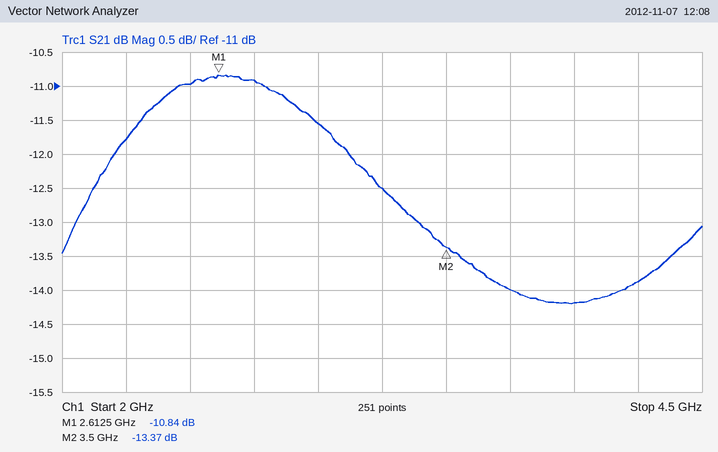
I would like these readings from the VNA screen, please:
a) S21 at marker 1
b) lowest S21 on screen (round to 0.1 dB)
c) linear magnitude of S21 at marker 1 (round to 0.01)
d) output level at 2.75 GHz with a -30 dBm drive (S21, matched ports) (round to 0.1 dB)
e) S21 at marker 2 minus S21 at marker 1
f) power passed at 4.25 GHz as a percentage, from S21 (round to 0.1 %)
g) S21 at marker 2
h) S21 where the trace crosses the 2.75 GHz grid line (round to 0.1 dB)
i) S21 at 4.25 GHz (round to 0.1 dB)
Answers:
-10.84 dB
-14.2 dB
0.29
-40.9 dBm
-2.53 dB
4.1 %
-13.37 dB
-10.9 dB
-13.9 dB
